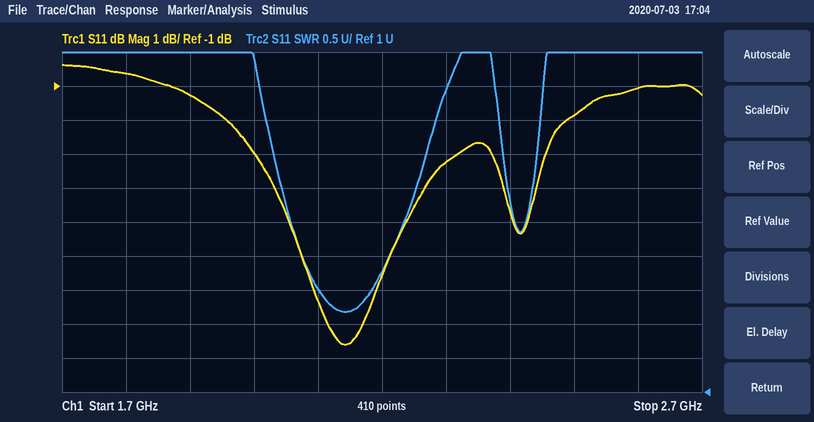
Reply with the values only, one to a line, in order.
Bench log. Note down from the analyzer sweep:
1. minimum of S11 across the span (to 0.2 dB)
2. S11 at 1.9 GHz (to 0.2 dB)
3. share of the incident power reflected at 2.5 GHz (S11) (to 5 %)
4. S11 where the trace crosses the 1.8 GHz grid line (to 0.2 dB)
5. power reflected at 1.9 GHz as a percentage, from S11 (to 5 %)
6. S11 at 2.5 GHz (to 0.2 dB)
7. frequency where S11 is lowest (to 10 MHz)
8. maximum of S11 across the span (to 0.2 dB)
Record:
-8.6 dB
-1.2 dB
65 %
-0.6 dB
75 %
-1.8 dB
2.14 GHz
-0.4 dB
